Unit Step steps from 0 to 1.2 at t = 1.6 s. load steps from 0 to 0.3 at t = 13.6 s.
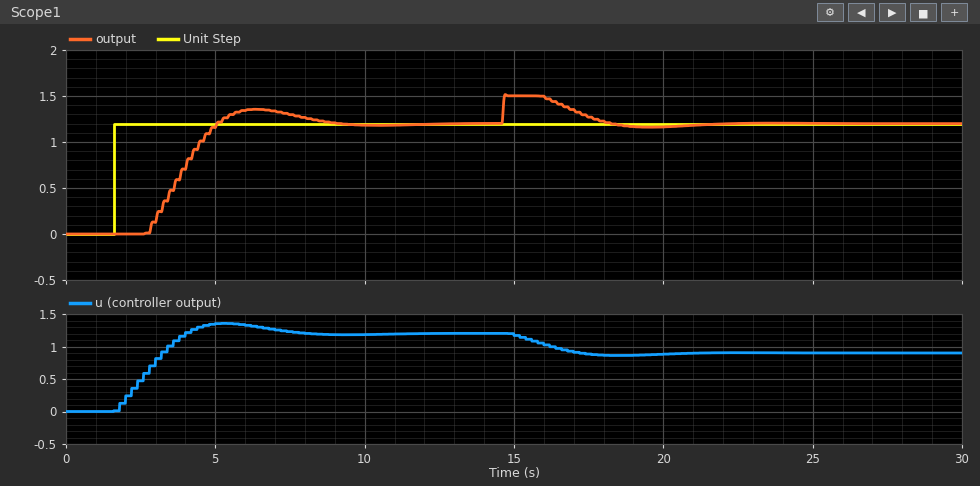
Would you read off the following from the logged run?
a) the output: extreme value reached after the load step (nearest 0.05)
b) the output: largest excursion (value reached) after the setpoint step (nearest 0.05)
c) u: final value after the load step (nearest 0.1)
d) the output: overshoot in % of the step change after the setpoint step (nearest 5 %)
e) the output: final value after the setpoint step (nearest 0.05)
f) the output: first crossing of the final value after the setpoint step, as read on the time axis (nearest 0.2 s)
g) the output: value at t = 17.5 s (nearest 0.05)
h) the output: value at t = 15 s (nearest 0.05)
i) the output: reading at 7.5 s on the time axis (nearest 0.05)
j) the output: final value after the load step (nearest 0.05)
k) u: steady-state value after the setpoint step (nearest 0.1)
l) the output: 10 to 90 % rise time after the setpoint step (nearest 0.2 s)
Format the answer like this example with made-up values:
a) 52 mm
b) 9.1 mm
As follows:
a) 1.50
b) 1.35
c) 0.9
d) 15 %
e) 1.20
f) 5.0 s
g) 1.25
h) 1.50
i) 1.30
j) 1.20
k) 1.2
l) 1.8 s
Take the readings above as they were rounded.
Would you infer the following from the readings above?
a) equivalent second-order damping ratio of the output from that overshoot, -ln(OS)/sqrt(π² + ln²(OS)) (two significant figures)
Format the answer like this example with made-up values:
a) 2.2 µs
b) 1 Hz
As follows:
a) 0.52
